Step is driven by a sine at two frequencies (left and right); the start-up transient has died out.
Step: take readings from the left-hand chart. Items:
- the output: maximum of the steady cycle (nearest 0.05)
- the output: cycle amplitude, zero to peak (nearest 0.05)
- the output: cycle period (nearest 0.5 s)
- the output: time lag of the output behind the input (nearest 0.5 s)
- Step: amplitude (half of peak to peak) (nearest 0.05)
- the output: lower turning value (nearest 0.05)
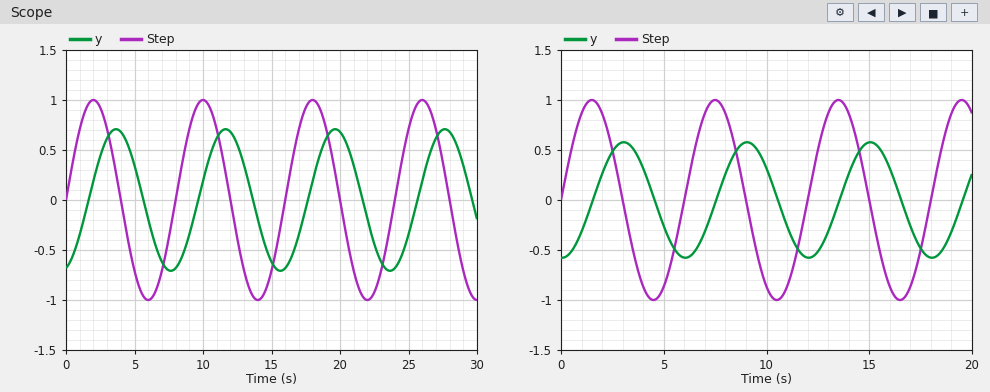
0.70
0.70
8.0 s
1.5 s
1.00
-0.70
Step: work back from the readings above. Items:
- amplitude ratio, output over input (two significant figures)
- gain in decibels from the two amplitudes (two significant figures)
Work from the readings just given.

0.70
-3.1 dB
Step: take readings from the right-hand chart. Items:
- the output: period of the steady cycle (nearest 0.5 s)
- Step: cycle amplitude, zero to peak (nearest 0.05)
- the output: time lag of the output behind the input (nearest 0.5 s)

6.0 s
1.00
1.5 s
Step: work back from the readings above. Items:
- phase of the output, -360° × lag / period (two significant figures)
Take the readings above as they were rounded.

-90°
